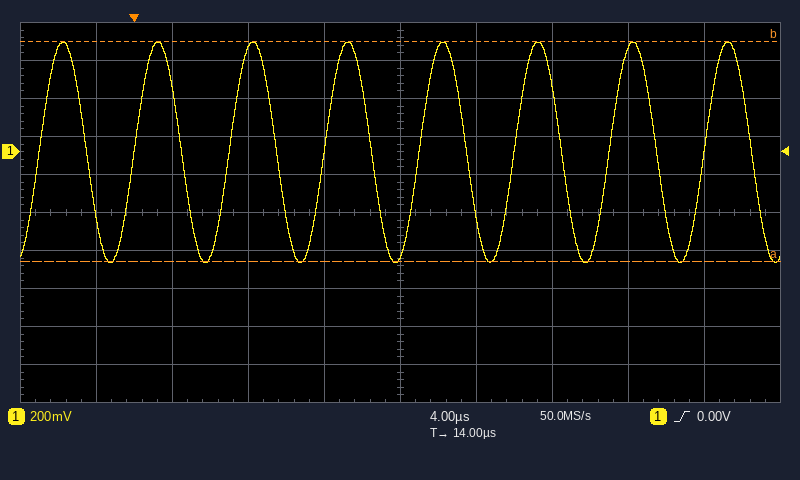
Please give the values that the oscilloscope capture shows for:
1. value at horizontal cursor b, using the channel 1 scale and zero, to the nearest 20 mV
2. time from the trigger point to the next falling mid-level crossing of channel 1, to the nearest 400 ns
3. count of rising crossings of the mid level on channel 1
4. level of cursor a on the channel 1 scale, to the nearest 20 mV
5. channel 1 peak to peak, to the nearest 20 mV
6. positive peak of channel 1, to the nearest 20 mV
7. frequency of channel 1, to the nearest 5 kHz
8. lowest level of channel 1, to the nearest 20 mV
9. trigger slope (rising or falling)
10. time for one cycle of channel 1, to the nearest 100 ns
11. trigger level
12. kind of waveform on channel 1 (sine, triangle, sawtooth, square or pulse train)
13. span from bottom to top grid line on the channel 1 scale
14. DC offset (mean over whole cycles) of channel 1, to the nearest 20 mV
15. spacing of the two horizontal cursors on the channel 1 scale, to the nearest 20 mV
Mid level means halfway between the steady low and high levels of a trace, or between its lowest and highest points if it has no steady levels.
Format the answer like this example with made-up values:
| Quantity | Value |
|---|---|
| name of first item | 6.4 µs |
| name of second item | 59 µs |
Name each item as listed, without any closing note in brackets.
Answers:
| Quantity | Value |
|---|---|
| value at horizontal cursor b, using the channel 1 scale and zero, to the nearest 20 mV | 580 mV |
| time from the trigger point to the next falling mid-level crossing of channel 1, to the nearest 400 ns | 2.4 µs |
| count of rising crossings of the mid level on channel 1 | 8 |
| level of cursor a on the channel 1 scale, to the nearest 20 mV | -580 mV |
| channel 1 peak to peak, to the nearest 20 mV | 1.16 V |
| positive peak of channel 1, to the nearest 20 mV | 580 mV |
| frequency of channel 1, to the nearest 5 kHz | 200 kHz |
| lowest level of channel 1, to the nearest 20 mV | -580 mV |
| trigger slope | rising |
| time for one cycle of channel 1, to the nearest 100 ns | 5.0 µs |
| trigger level | 0.00 V |
| kind of waveform on channel 1 | sine |
| span from bottom to top grid line on the channel 1 scale | 2 V |
| DC offset (mean over whole cycles) of channel 1, to the nearest 20 mV | 0 mV |
| spacing of the two horizontal cursors on the channel 1 scale, to the nearest 20 mV | 1.16 V |
